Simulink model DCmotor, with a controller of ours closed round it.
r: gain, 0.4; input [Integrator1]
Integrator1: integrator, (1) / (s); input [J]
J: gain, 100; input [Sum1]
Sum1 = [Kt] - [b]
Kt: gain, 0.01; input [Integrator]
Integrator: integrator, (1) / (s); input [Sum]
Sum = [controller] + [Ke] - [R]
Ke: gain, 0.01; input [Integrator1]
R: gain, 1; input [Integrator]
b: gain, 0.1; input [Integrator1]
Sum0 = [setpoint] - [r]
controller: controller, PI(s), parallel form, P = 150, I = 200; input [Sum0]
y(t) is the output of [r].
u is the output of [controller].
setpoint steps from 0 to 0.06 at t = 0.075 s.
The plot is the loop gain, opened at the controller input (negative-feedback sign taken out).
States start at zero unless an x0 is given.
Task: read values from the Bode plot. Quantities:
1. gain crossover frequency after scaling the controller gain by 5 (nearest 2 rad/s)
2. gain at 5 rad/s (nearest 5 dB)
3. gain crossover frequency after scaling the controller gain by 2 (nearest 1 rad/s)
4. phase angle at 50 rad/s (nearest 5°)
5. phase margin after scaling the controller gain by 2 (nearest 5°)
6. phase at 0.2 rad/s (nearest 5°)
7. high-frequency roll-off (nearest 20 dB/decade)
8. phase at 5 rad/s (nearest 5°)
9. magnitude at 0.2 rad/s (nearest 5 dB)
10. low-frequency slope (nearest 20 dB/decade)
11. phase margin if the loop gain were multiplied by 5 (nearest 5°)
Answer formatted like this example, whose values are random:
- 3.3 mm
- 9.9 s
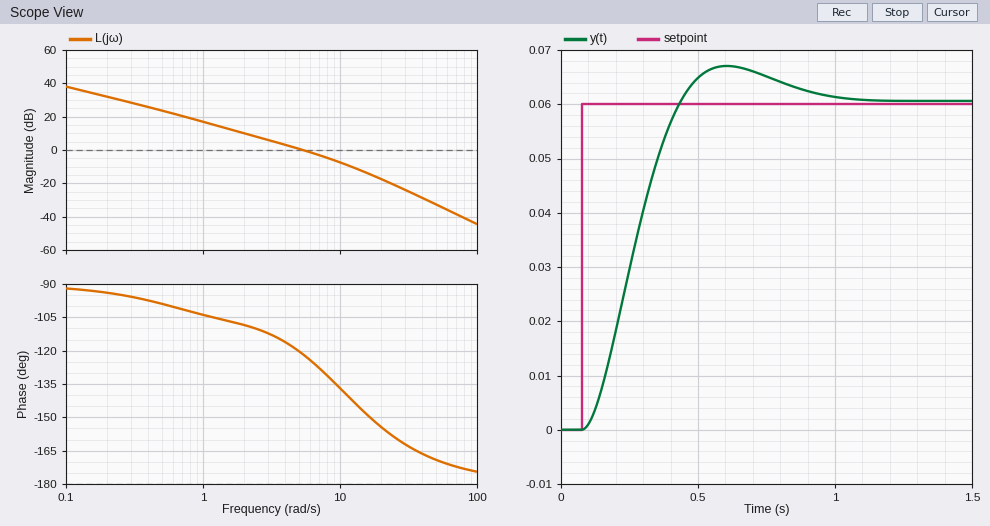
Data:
- 16 rad/s
- 0 dB
- 9 rad/s
- -170°
- 45°
- -95°
- -40 dB/decade
- -120°
- 30 dB
- -20 dB/decade
- 30°
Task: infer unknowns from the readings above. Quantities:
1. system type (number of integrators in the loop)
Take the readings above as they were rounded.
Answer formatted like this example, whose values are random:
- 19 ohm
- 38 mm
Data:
- 1
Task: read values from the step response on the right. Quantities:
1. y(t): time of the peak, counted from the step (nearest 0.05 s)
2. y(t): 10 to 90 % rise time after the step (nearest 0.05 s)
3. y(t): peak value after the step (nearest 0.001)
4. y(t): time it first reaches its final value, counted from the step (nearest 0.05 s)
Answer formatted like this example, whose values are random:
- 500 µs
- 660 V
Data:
- 0.55 s
- 0.25 s
- 0.067
- 0.35 s
